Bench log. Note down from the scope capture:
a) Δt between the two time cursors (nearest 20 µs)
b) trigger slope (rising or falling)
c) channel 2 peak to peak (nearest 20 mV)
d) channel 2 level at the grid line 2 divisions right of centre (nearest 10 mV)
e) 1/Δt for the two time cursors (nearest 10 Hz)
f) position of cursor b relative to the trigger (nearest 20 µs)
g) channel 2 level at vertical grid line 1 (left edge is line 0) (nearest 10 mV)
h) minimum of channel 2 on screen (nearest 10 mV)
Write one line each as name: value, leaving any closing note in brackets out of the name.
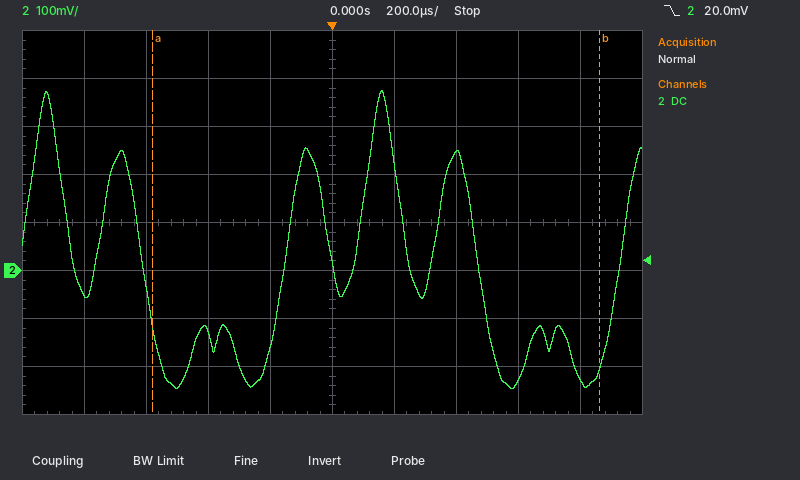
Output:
Δt between the two time cursors: 1.44 ms
trigger slope: falling
channel 2 peak to peak: 620 mV
channel 2 level at the grid line 2 divisions right of centre: 240 mV
1/Δt for the two time cursors: 690 Hz
position of cursor b relative to the trigger: +860 µs
channel 2 level at vertical grid line 1 (left edge is line 0): -50 mV
minimum of channel 2 on screen: -250 mV
